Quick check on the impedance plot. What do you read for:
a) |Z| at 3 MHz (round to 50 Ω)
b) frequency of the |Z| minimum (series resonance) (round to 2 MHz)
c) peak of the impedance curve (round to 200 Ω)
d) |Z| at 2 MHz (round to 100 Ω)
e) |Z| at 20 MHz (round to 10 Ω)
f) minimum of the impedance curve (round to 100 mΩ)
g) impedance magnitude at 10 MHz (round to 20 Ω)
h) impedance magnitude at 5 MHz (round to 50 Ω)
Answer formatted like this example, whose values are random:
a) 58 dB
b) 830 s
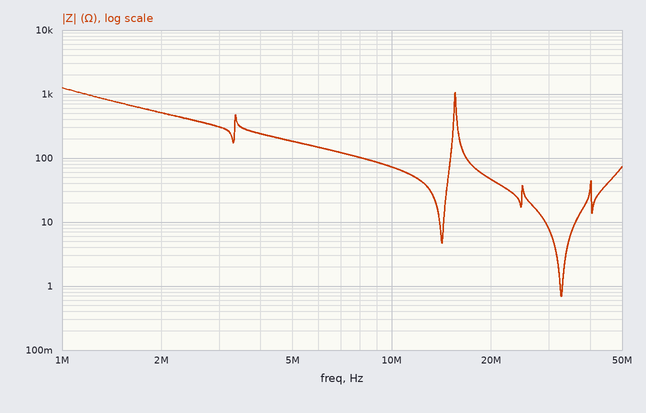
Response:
a) 300 Ω
b) 32 MHz
c) 1.2 kΩ
d) 500 Ω
e) 50 Ω
f) 700 mΩ
g) 80 Ω
h) 200 Ω
